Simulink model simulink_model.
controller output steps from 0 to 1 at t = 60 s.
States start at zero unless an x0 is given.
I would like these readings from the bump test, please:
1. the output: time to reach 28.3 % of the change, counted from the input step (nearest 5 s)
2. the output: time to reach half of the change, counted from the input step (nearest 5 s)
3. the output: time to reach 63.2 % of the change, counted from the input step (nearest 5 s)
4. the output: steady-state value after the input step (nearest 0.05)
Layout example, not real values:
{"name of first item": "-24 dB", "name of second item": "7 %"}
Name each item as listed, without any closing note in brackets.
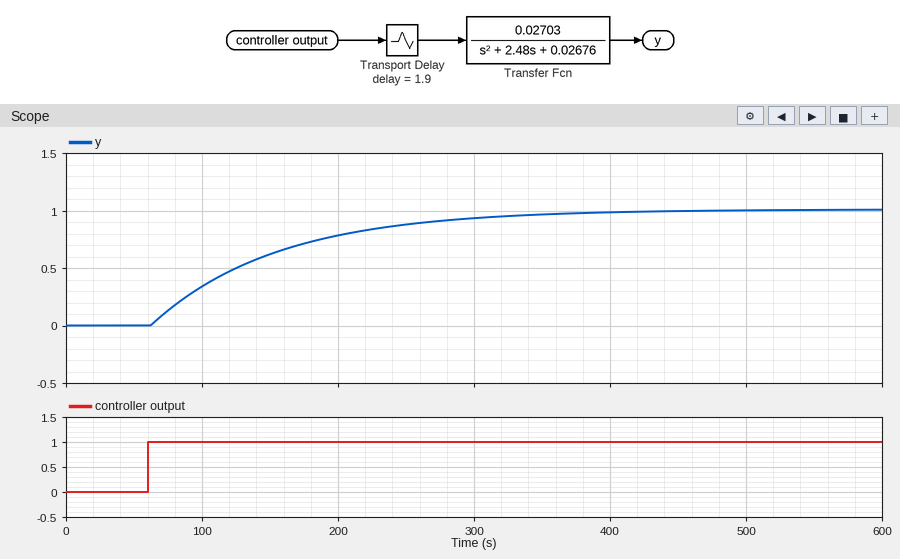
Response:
{"the output: time to reach 28.3 % of the change, counted from the input step": "35 s", "the output: time to reach half of the change, counted from the input step": "65 s", "the output: time to reach 63.2 % of the change, counted from the input step": "95 s", "the output: steady-state value after the input step": "1.00"}
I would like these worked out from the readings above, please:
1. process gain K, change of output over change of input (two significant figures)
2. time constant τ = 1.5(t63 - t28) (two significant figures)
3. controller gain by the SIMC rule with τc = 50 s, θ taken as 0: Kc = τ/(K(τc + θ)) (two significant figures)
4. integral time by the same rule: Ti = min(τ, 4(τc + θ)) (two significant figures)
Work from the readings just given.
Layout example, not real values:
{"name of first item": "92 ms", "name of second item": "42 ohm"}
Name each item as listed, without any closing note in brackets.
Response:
{"process gain K, change of output over change of input": "1.0", "time constant τ = 1.5(t63 - t28)": "90 s", "controller gain by the SIMC rule with τc = 50 s, θ taken as 0: Kc = τ/(K(τc + θ))": "1.8", "integral time by the same rule: Ti = min(τ, 4(τc + θ))": "90 s"}
